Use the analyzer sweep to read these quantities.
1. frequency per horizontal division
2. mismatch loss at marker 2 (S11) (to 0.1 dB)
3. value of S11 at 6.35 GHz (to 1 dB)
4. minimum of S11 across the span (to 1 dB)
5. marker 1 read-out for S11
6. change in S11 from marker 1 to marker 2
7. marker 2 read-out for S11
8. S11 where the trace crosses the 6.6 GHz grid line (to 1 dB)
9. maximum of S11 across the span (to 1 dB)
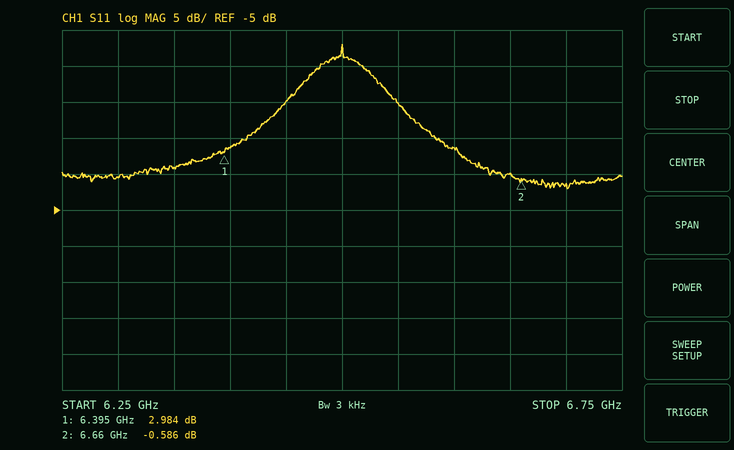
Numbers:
50 MHz
9.0 dB
1 dB
-2 dB
2.984 dB
-3.570 dB
-0.586 dB
4 dB
18 dB
